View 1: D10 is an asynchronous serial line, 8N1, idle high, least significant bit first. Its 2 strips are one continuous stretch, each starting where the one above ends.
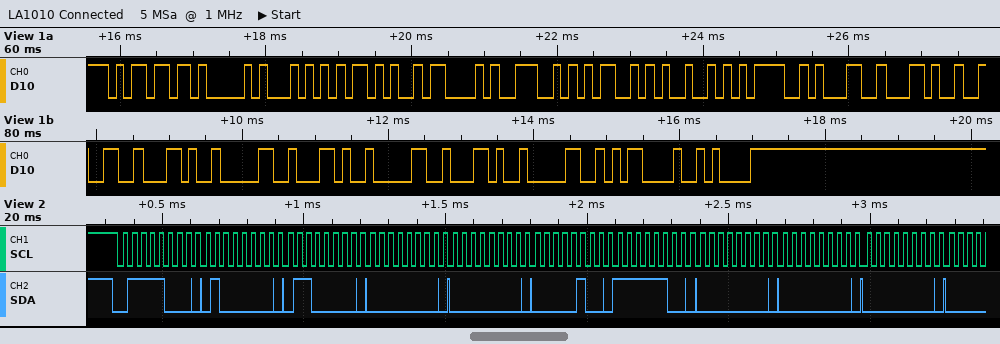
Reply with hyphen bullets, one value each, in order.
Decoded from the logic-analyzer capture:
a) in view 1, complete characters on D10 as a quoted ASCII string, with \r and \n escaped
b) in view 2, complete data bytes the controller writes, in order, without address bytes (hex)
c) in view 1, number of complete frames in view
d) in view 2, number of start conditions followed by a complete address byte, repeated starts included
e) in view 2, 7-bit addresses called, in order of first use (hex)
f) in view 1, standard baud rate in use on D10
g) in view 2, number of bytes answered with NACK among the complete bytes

- "mAT+CNMI=1,2,0,0,0\r\n"
- 40 60 00 00 04 FC 00 00 00
- 20
- 1
- 0x3C
- 9600 baud
- 0
